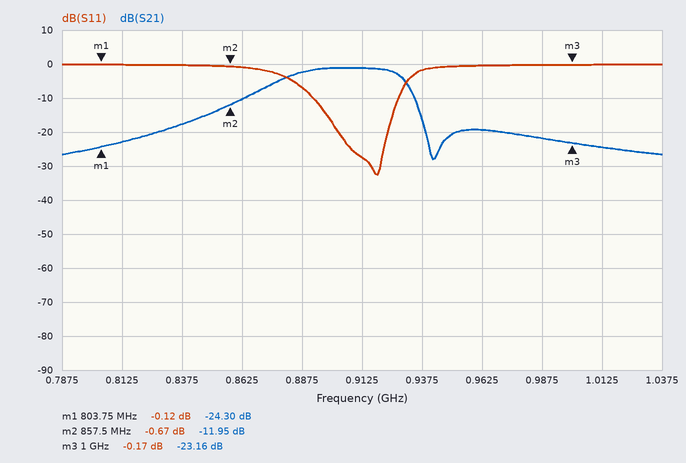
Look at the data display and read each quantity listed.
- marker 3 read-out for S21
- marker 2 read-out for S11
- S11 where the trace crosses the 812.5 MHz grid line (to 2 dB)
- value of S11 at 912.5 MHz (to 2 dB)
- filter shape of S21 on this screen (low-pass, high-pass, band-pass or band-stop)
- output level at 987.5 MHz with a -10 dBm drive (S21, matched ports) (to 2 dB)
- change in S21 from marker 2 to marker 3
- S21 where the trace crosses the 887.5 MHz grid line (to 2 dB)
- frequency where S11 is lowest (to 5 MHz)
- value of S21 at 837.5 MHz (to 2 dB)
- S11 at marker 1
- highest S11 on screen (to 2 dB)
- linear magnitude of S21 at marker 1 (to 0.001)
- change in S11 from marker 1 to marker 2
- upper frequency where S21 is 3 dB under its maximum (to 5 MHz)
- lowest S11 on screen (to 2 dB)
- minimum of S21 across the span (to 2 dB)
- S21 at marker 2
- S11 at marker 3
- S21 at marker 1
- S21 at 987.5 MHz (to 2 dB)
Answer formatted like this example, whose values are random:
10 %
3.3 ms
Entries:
-23.16 dB
-0.67 dB
0 dB
-28 dB
band-pass
-32 dBm
-11.21 dB
-2 dB
920 MHz
-18 dB
-0.12 dB
0 dB
0.061
-0.55 dB
930 MHz
-32 dB
-28 dB
-11.95 dB
-0.17 dB
-24.30 dB
-22 dB
